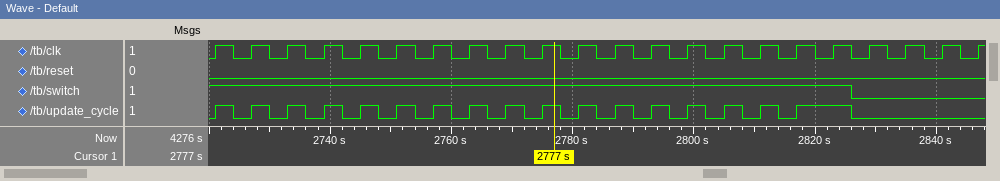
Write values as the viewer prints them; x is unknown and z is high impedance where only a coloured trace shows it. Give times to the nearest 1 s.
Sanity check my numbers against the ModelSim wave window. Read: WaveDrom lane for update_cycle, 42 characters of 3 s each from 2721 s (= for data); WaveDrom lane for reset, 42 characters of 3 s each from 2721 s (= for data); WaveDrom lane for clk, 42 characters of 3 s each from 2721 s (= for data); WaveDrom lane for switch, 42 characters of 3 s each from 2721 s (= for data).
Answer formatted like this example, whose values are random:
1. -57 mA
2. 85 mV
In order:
1. {name: 'update_cycle', wave: '101010101010101010101010101010101..0......'}
2. {name: 'reset', wave: '0.........................................'}
3. {name: 'clk', wave: '101010101010101010101010101010101010101010'}
4. {name: 'switch', wave: '1..................................0......'}
